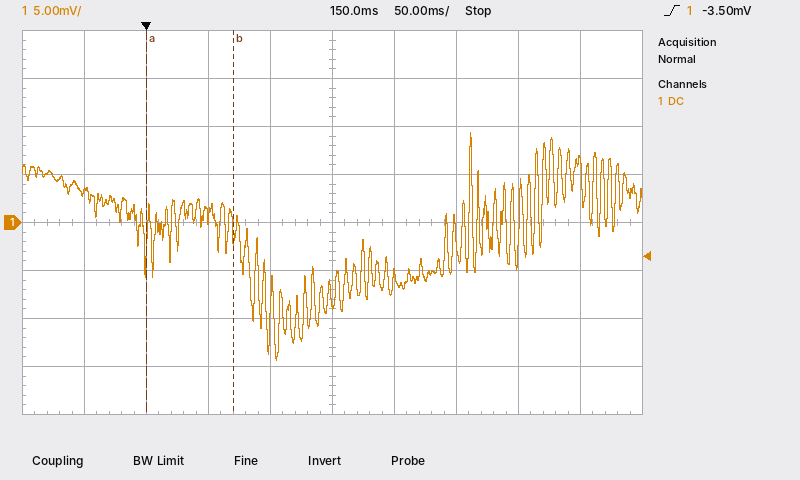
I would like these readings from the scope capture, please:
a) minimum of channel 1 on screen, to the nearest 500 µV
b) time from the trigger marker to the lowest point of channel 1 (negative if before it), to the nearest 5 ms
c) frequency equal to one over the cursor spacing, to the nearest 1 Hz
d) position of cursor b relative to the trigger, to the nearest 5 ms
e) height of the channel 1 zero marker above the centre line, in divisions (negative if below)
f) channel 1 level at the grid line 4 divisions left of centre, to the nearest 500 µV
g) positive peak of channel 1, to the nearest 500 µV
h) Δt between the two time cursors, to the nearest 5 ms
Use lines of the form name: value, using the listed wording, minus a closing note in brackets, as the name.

minimum of channel 1 on screen, to the nearest 500 µV: -14.5 mV
time from the trigger marker to the lowest point of channel 1 (negative if before it), to the nearest 5 ms: +105 ms
frequency equal to one over the cursor spacing, to the nearest 1 Hz: 14 Hz
position of cursor b relative to the trigger, to the nearest 5 ms: +70 ms
height of the channel 1 zero marker above the centre line, in divisions: 0.0 div
channel 1 level at the grid line 4 divisions left of centre, to the nearest 500 µV: 3.0 mV
positive peak of channel 1, to the nearest 500 µV: 9.5 mV
Δt between the two time cursors, to the nearest 5 ms: 70 ms
